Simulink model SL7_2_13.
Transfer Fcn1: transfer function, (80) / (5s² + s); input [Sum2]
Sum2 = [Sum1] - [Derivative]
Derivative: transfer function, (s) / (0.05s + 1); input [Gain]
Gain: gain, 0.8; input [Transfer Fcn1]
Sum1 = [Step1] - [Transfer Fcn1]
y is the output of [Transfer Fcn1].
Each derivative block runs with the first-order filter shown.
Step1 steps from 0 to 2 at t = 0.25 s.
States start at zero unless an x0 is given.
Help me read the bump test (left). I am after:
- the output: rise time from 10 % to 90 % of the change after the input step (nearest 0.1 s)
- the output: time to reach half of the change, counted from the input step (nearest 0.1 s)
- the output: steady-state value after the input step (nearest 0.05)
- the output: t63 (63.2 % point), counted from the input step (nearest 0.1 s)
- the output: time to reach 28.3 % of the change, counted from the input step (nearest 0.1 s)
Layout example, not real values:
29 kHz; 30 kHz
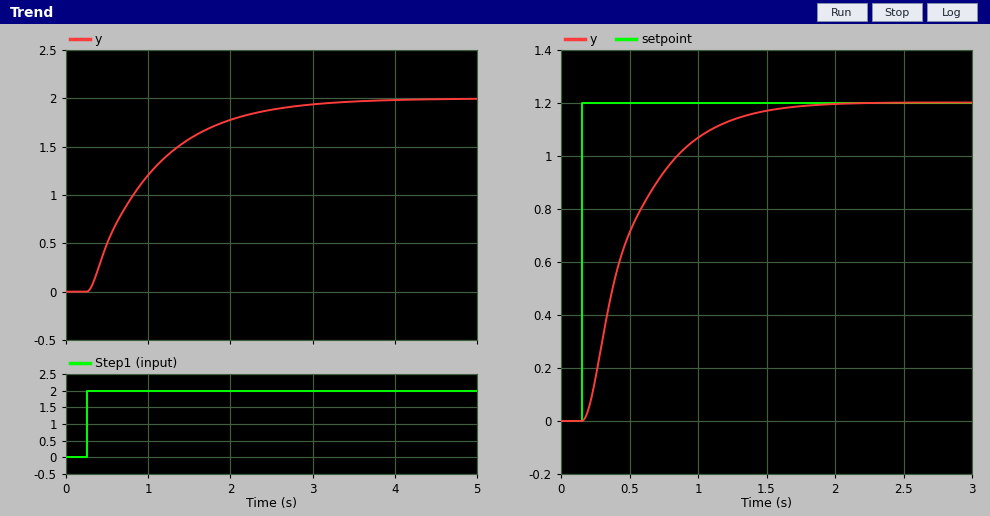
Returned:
1.7 s; 0.6 s; 2.00; 0.8 s; 0.3 s
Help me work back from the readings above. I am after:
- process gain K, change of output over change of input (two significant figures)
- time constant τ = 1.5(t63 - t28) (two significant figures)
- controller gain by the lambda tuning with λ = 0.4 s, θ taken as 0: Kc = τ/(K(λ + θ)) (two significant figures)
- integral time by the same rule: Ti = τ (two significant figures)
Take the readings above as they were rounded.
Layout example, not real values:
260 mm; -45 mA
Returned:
1.0; 0.75 s; 1.9; 0.75 s
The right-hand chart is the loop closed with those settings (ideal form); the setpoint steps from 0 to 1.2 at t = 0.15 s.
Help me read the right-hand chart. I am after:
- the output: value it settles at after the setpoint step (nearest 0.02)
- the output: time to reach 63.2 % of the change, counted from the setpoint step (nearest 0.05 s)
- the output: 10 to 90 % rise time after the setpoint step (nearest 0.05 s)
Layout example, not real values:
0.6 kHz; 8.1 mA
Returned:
1.20; 0.40 s; 0.80 s
